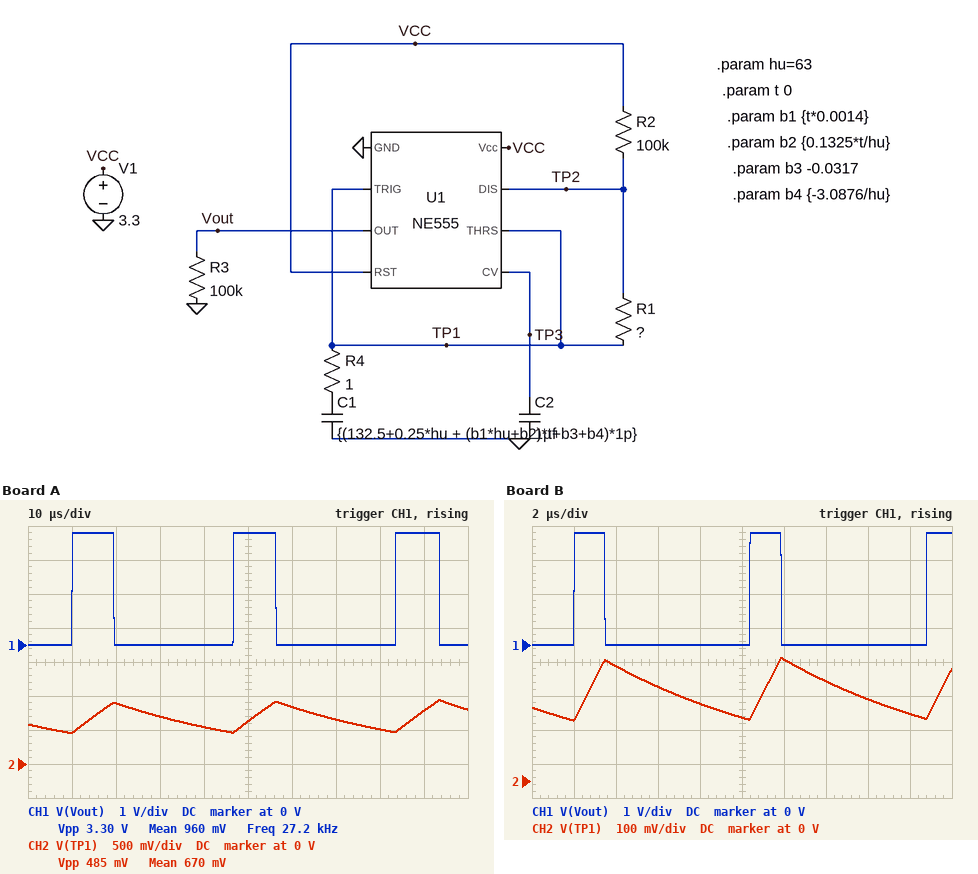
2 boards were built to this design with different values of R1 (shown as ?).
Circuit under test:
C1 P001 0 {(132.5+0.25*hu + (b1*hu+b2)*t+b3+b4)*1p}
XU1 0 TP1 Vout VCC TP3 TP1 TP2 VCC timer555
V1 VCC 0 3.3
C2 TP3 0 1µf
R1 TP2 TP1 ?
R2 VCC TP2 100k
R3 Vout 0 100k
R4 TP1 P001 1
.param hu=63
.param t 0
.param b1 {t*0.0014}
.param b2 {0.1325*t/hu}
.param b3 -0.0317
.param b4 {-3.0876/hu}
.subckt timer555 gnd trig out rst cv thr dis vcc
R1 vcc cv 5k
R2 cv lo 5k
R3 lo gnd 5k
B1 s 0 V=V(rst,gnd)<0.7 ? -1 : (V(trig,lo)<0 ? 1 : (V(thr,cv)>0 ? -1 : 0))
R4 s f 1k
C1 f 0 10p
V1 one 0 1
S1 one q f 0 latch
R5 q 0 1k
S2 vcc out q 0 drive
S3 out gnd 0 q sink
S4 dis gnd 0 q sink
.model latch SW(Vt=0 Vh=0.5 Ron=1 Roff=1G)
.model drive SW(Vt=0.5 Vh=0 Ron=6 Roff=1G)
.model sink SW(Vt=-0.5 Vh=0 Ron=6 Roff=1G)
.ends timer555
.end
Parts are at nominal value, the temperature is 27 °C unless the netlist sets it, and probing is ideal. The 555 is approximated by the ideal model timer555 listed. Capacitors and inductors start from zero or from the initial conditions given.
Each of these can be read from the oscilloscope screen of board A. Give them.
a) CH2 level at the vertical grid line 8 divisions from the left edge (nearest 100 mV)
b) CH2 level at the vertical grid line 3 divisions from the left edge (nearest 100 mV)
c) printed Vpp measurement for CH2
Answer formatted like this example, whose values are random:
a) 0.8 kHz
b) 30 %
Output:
a) 500 mV
b) 700 mV
c) 485 mV
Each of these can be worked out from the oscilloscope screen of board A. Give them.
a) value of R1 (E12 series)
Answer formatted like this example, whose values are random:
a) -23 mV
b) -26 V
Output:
a) 270 kΩ
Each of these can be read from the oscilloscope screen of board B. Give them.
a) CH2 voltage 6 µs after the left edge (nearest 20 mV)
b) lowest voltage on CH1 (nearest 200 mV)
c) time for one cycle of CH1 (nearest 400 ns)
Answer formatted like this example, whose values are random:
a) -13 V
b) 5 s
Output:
a) 280 mV
b) 0 V
c) 8.4 µs
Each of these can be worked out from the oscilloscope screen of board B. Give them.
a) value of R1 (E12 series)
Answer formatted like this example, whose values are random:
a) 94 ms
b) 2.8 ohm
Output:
a) 68 kΩ
